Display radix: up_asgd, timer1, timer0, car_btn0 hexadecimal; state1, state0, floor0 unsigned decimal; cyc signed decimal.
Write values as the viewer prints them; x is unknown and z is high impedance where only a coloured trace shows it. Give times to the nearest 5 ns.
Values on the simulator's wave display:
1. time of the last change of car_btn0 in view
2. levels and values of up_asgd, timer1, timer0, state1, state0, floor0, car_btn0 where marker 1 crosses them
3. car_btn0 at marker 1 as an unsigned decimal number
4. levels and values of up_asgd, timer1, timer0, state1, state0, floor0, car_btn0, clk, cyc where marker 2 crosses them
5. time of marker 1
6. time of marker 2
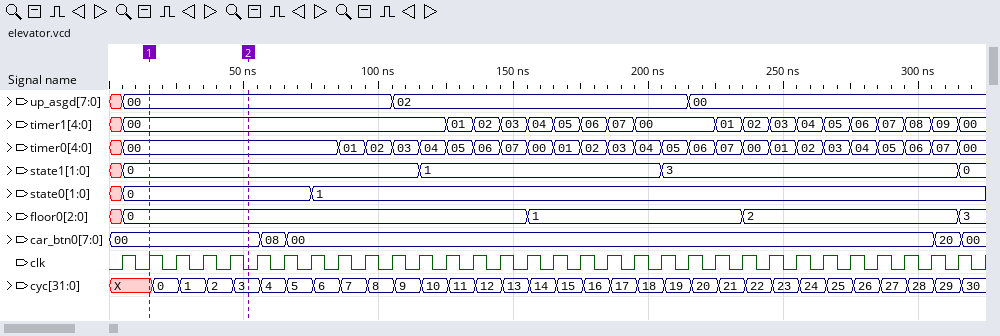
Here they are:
315 ns
up_asgd=00, timer1=00, timer0=00, state1=0, state0=0, floor0=0, car_btn0=00
0
up_asgd=00, timer1=00, timer0=00, state1=0, state0=0, floor0=0, car_btn0=00, clk=0, cyc=3
15 ns
50 ns
